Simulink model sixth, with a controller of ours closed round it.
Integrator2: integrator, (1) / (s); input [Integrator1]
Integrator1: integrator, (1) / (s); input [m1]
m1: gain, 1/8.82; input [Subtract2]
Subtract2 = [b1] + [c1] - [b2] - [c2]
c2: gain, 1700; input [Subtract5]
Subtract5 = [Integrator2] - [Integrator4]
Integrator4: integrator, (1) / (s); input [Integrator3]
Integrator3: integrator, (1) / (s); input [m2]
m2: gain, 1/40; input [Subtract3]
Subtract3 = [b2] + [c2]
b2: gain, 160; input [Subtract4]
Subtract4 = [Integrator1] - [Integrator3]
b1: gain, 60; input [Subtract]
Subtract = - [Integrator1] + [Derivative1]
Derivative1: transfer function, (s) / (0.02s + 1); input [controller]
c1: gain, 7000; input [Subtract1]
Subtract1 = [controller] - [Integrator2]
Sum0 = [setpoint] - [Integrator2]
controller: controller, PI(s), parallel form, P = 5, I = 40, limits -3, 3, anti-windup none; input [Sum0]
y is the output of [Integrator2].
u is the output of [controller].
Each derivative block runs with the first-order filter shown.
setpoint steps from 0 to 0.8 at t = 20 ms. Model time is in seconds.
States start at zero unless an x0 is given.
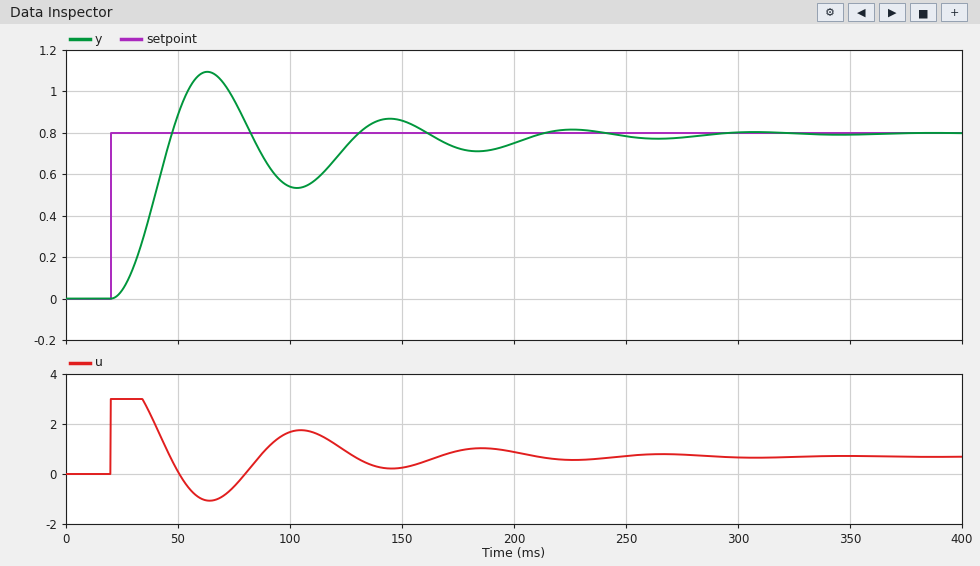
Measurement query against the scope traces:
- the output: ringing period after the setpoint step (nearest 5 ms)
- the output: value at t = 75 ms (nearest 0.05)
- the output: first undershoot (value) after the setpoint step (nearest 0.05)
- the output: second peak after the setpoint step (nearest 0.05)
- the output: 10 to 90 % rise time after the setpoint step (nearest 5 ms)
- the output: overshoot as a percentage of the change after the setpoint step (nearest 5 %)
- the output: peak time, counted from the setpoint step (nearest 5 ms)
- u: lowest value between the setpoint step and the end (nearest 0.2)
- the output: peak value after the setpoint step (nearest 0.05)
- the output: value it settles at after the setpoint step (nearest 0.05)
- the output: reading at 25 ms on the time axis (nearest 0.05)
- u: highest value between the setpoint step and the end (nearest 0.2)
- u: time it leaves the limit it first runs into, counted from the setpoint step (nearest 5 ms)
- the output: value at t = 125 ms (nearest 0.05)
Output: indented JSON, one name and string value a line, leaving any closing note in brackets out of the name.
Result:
{
  "the output: ringing period after the setpoint step": "80 ms",
  "the output: value at t = 75 ms": "0.95",
  "the output: first undershoot (value) after the setpoint step": "0.55",
  "the output: second peak after the setpoint step": "0.85",
  "the output: 10 to 90 % rise time after the setpoint step": "20 ms",
  "the output: overshoot as a percentage of the change after the setpoint step": "35 %",
  "the output: peak time, counted from the setpoint step": "45 ms",
  "u: lowest value between the setpoint step and the end": "-1.0",
  "the output: peak value after the setpoint step": "1.10",
  "the output: value it settles at after the setpoint step": "0.80",
  "the output: reading at 25 ms on the time axis": "0.05",
  "u: highest value between the setpoint step and the end": "3.0",
  "u: time it leaves the limit it first runs into, counted from the setpoint step": "15 ms",
  "the output: value at t = 125 ms": "0.75"
}
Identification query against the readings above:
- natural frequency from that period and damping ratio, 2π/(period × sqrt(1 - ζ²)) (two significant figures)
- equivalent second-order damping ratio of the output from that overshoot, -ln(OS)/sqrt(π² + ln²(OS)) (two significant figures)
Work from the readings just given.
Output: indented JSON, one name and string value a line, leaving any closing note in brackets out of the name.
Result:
{
  "natural frequency from that period and damping ratio, 2π/(period × sqrt(1 - ζ²))": "0.083 rad/ms",
  "equivalent second-order damping ratio of the output from that overshoot, -ln(OS)/sqrt(π² + ln²(OS))": "0.32"
}
